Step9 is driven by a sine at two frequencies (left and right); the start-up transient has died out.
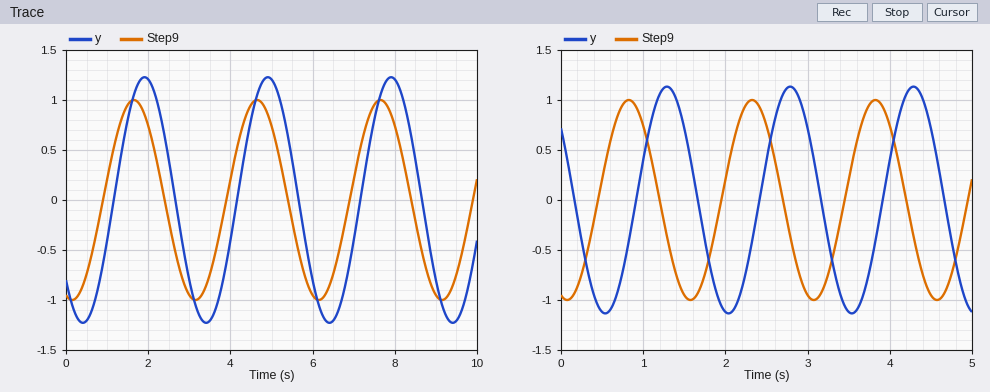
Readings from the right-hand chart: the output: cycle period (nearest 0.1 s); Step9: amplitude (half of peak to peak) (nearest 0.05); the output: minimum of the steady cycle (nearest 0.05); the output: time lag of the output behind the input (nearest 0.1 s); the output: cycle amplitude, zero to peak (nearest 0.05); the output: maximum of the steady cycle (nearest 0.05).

1.5 s
1.00
-1.15
0.5 s
1.15
1.15
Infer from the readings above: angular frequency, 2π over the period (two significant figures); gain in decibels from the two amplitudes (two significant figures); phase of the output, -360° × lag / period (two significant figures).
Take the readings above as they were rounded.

4.2 rad/s
1.2 dB
-120°
